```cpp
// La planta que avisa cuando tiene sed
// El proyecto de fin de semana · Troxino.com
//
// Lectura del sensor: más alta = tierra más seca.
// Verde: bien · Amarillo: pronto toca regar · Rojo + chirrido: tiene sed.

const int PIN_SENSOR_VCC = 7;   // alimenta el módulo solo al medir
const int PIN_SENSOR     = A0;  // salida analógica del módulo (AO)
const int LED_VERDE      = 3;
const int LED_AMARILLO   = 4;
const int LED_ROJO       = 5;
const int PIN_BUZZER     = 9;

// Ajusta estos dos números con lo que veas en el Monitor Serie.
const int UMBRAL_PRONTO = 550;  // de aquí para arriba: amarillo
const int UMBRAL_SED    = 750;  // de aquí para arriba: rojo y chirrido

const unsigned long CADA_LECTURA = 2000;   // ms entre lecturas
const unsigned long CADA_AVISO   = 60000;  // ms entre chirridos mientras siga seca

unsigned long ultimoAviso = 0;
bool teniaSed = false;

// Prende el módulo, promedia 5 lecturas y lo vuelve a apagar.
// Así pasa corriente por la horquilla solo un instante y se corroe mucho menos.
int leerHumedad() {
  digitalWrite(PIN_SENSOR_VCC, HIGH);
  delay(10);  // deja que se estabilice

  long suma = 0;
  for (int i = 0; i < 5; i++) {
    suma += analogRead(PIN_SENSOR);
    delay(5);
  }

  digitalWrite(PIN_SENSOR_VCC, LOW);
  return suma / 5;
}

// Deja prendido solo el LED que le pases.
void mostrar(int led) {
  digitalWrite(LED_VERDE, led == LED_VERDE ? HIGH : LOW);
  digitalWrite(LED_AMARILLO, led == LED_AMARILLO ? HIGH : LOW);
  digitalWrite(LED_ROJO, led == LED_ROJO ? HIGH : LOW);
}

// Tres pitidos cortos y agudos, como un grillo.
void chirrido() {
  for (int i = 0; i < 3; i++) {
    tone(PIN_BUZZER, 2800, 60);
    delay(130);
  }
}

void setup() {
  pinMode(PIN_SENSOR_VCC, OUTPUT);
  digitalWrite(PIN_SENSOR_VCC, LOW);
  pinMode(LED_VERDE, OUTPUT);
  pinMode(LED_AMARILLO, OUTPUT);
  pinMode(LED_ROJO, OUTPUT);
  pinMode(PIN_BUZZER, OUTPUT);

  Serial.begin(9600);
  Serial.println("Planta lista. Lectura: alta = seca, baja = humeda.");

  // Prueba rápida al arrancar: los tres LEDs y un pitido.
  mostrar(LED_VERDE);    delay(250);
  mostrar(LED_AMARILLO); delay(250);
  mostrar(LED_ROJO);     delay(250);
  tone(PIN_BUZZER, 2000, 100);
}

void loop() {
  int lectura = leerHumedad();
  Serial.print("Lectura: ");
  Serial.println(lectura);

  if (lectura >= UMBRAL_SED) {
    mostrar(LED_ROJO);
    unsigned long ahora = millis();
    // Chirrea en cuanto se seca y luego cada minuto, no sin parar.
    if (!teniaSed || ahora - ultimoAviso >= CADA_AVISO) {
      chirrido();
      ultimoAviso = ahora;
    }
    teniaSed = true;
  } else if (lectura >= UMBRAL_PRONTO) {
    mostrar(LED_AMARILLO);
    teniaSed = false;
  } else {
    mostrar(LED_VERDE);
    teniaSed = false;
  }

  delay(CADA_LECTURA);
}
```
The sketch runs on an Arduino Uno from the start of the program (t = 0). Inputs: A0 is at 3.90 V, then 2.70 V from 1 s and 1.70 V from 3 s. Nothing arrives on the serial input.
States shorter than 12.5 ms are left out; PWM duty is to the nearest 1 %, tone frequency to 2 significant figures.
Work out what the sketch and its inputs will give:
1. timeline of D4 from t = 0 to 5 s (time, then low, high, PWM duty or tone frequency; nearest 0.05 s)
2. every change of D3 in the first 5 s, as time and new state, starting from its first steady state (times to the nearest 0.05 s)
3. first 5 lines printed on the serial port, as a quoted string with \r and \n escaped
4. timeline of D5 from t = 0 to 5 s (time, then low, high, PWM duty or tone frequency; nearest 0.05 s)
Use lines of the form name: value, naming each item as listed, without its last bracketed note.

timeline of D4 from t = 0 to 5 s: 0 s low; 0.25 s high; 0.5 s low
every change of D3 in the first 5 s, as time and new state, starting from its first steady state: 0 s high; 0.25 s low; 3.2 s high
first 5 lines printed on the serial port, as a quoted string with \r and \n escaped: "Planta lista. Lectura: alta = seca, baja = humeda.\r\nLectura: 798\r\nLectura: 348\r\nLectura: 348\r\nLectura: 348\r\n"
timeline of D5 from t = 0 to 5 s: 0 s low; 0.5 s high; 3.2 s low
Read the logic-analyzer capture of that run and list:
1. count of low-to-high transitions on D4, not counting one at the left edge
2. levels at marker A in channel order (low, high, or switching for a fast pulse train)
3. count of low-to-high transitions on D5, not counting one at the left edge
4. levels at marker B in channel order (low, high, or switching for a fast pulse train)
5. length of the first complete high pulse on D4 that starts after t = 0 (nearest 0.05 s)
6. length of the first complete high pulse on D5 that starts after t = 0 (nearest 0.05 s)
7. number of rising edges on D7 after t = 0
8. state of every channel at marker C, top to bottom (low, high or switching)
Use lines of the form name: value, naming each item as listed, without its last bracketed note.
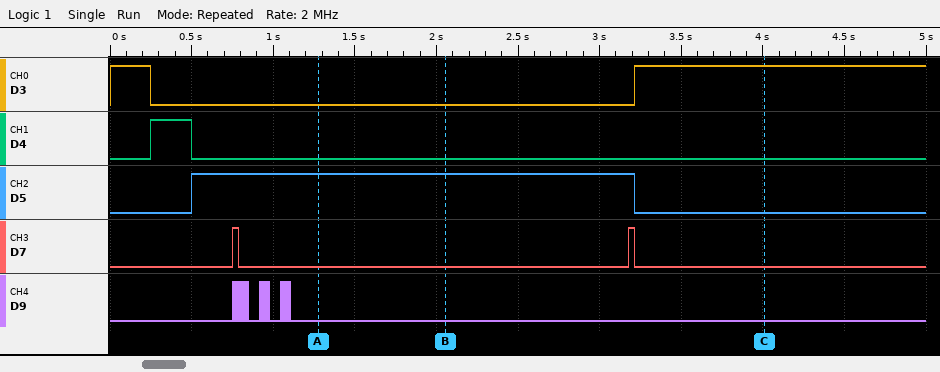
count of low-to-high transitions on D4, not counting one at the left edge: 1
levels at marker A in channel order: D3 low, D4 low, D5 high, D7 low, D9 low
count of low-to-high transitions on D5, not counting one at the left edge: 1
levels at marker B in channel order: D3 low, D4 low, D5 high, D7 low, D9 low
length of the first complete high pulse on D4 that starts after t = 0: 0.25 s
length of the first complete high pulse on D5 that starts after t = 0: 2.70 s
number of rising edges on D7 after t = 0: 2
state of every channel at marker C, top to bottom: D3 high, D4 low, D5 low, D7 low, D9 low
